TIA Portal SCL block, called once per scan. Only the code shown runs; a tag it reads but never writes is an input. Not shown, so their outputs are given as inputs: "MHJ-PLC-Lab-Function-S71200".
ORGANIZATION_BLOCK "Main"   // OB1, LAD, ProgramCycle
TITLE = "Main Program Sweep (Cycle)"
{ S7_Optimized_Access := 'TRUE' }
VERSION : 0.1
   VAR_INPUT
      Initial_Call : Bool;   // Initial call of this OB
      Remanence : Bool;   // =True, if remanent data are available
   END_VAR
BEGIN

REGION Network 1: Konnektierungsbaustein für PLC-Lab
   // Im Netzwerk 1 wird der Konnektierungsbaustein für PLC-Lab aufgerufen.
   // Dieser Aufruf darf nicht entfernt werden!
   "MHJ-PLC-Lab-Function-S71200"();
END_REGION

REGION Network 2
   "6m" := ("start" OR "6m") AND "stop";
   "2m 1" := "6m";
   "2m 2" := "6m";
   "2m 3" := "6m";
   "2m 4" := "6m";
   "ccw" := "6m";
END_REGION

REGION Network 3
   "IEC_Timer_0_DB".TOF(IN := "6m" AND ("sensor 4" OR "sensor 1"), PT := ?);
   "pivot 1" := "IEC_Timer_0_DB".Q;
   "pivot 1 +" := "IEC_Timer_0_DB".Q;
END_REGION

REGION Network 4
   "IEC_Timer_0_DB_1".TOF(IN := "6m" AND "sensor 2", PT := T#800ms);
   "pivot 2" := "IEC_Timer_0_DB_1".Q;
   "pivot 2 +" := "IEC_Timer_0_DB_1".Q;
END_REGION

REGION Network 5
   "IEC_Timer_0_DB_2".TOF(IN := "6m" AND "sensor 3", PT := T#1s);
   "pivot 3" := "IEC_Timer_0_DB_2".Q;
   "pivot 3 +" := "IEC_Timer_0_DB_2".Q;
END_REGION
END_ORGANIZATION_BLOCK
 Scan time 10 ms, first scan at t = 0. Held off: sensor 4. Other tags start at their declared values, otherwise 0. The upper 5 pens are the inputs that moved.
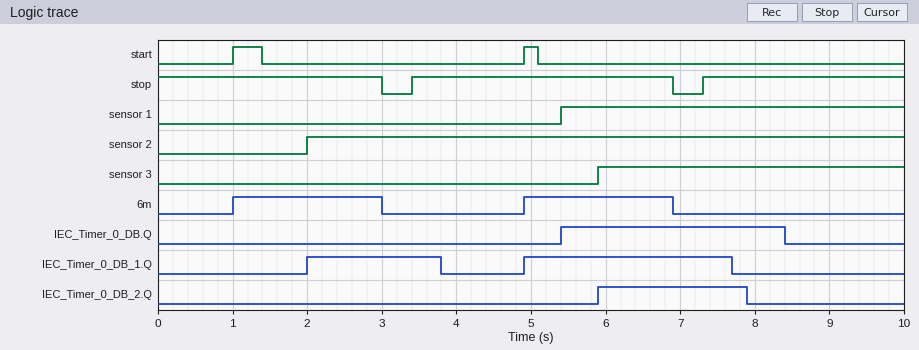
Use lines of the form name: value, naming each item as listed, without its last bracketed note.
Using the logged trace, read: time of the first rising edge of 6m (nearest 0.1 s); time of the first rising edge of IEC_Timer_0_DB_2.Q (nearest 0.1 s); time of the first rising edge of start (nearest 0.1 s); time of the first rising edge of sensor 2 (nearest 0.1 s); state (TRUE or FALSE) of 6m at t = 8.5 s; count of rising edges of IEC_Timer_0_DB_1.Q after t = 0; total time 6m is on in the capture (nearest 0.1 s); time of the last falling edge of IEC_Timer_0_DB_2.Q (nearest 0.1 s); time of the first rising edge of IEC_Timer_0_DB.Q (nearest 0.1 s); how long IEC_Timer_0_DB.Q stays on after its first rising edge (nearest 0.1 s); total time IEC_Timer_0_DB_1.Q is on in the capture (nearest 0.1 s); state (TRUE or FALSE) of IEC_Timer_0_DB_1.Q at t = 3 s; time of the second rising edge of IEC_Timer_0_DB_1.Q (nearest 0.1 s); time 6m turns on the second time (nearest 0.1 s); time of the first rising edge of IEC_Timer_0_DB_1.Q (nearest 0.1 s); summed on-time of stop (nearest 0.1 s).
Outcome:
time of the first rising edge of 6m: 1.0 s
time of the first rising edge of IEC_Timer_0_DB_2.Q: 5.9 s
time of the first rising edge of start: 1.0 s
time of the first rising edge of sensor 2: 2.0 s
state (TRUE or FALSE) of 6m at t = 8.5 s: FALSE
count of rising edges of IEC_Timer_0_DB_1.Q after t = 0: 2
total time 6m is on in the capture: 4.0 s
time of the last falling edge of IEC_Timer_0_DB_2.Q: 7.9 s
time of the first rising edge of IEC_Timer_0_DB.Q: 5.4 s
how long IEC_Timer_0_DB.Q stays on after its first rising edge: 3.0 s
total time IEC_Timer_0_DB_1.Q is on in the capture: 4.6 s
state (TRUE or FALSE) of IEC_Timer_0_DB_1.Q at t = 3 s: TRUE
time of the second rising edge of IEC_Timer_0_DB_1.Q: 4.9 s
time 6m turns on the second time: 4.9 s
time of the first rising edge of IEC_Timer_0_DB_1.Q: 2.0 s
summed on-time of stop: 9.2 s
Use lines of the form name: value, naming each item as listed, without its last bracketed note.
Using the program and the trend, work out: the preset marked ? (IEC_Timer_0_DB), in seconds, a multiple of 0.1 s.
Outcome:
the preset marked ? (IEC_Timer_0_DB), in seconds, a multiple of 0.1 s: 1.5 s
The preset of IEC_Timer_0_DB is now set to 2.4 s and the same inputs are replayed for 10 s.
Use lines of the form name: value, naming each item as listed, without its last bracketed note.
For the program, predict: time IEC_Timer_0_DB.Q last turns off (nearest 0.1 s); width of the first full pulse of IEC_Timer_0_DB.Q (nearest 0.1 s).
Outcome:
time IEC_Timer_0_DB.Q last turns off: 9.3 s
width of the first full pulse of IEC_Timer_0_DB.Q: 3.9 s
